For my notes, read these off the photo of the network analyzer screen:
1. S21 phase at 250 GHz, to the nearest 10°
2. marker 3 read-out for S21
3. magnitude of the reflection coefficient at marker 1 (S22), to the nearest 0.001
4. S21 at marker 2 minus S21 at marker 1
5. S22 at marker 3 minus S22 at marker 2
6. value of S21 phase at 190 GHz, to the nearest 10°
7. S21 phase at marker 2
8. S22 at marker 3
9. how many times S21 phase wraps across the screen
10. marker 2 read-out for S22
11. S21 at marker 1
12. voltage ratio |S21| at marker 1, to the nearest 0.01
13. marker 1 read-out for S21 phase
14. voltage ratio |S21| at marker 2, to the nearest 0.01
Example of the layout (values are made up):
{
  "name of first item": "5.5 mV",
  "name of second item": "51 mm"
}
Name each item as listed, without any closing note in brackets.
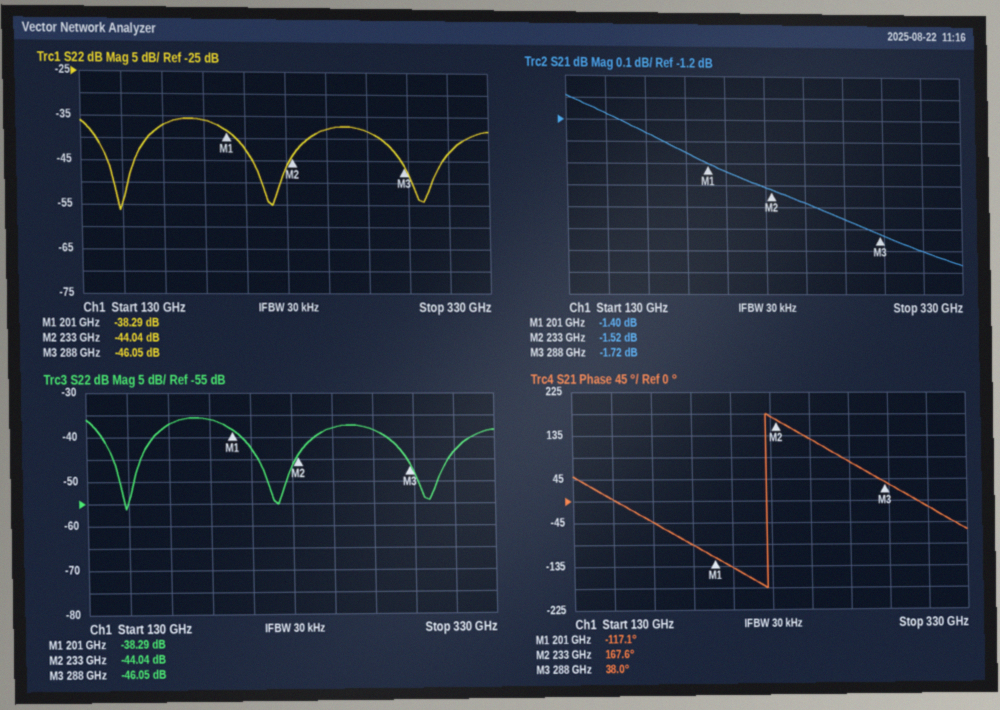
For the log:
{
  "S21 phase at 250 GHz, to the nearest 10°": "130°",
  "marker 3 read-out for S21": "-1.72 dB",
  "magnitude of the reflection coefficient at marker 1 (S22), to the nearest 0.001": "0.012",
  "S21 at marker 2 minus S21 at marker 1": "-0.12 dB",
  "S22 at marker 3 minus S22 at marker 2": "-2.01 dB",
  "value of S21 phase at 190 GHz, to the nearest 10°": "-90°",
  "S21 phase at marker 2": "167.6°",
  "S22 at marker 3": "-46.05 dB",
  "how many times S21 phase wraps across the screen": "1",
  "marker 2 read-out for S22": "-44.04 dB",
  "S21 at marker 1": "-1.40 dB",
  "voltage ratio |S21| at marker 1, to the nearest 0.01": "0.85",
  "marker 1 read-out for S21 phase": "-117.1°",
  "voltage ratio |S21| at marker 2, to the nearest 0.01": "0.84"
}
